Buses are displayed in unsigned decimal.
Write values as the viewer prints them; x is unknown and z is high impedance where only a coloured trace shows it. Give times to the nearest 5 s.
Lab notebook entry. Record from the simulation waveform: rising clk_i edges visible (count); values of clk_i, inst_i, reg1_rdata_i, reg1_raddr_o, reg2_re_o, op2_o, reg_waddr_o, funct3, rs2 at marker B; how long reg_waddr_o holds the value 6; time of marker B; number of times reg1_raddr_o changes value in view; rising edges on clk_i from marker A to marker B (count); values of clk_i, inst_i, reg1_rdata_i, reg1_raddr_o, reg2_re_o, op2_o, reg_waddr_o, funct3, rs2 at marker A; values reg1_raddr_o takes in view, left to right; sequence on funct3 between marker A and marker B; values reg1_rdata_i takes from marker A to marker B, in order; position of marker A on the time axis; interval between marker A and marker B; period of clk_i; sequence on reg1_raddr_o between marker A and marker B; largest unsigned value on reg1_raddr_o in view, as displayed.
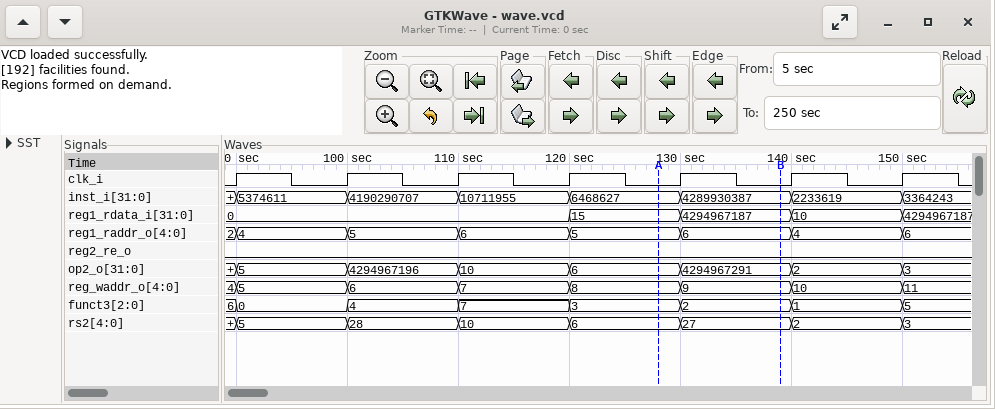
7
clk_i=0, inst_i=4289930387, reg1_rdata_i=4294967187, reg1_raddr_o=6, reg2_re_o=0, op2_o=4294967291, reg_waddr_o=9, funct3=2, rs2=27
10 s
140 s
7
1
clk_i=0, inst_i=6468627, reg1_rdata_i=15, reg1_raddr_o=5, reg2_re_o=0, op2_o=6, reg_waddr_o=8, funct3=3, rs2=6
2, 4, 5, 6, 5, 6, 4, 6
3, 2
15, 4294967187
130 s
10 s
10 s
5, 6
6
